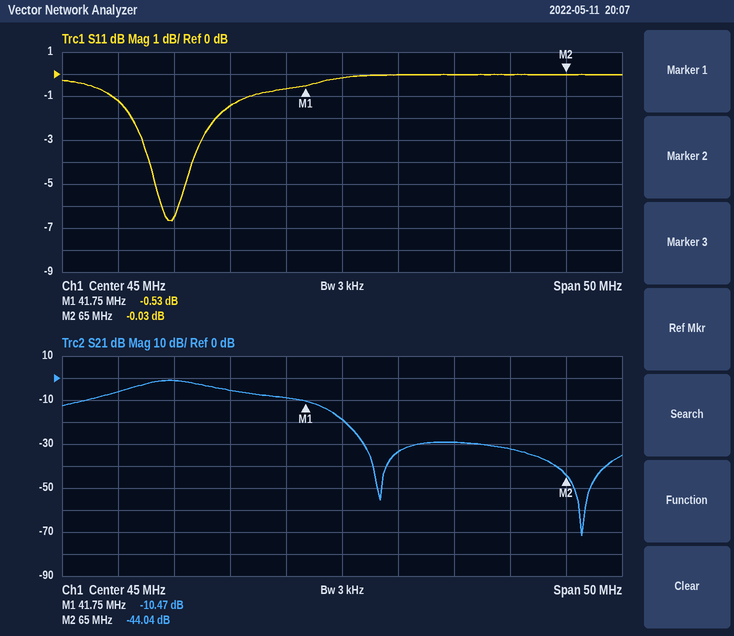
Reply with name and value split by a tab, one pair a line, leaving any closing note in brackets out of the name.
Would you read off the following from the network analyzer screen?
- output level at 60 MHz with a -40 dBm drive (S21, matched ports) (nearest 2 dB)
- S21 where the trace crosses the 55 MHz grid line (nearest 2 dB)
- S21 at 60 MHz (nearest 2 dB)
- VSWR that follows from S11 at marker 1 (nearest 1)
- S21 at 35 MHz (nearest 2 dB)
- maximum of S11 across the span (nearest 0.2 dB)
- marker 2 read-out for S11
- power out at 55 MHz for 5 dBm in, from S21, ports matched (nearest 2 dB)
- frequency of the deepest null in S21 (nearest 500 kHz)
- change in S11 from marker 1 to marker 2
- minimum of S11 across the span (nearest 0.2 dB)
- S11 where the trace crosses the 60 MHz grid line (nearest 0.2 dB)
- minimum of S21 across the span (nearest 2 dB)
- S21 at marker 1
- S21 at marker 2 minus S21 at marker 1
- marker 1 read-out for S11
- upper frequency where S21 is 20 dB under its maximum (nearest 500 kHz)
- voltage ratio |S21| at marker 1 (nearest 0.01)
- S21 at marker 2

output level at 60 MHz with a -40 dBm drive (S21, matched ports)	-72 dBm
S21 where the trace crosses the 55 MHz grid line	-30 dB
S21 at 60 MHz	-32 dB
VSWR that follows from S11 at marker 1	33
S21 at 35 MHz	-6 dB
maximum of S11 across the span	0.0 dB
marker 2 read-out for S11	-0.03 dB
power out at 55 MHz for 5 dBm in, from S21, ports matched	-24 dBm
frequency of the deepest null in S21	66.5 MHz
change in S11 from marker 1 to marker 2	0.50 dB
minimum of S11 across the span	-6.6 dB
S11 where the trace crosses the 60 MHz grid line	0.0 dB
minimum of S21 across the span	-72 dB
S21 at marker 1	-10.47 dB
S21 at marker 2 minus S21 at marker 1	-33.57 dB
marker 1 read-out for S11	-0.53 dB
upper frequency where S21 is 20 dB under its maximum	45.5 MHz
voltage ratio |S21| at marker 1	0.30
S21 at marker 2	-44.04 dB
